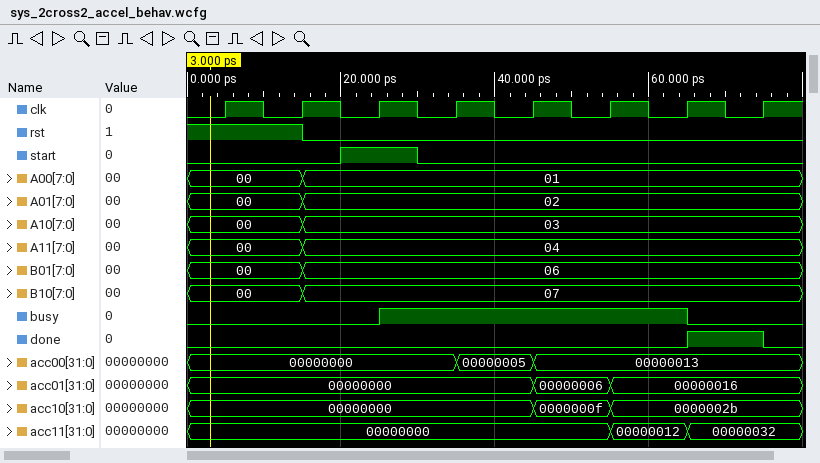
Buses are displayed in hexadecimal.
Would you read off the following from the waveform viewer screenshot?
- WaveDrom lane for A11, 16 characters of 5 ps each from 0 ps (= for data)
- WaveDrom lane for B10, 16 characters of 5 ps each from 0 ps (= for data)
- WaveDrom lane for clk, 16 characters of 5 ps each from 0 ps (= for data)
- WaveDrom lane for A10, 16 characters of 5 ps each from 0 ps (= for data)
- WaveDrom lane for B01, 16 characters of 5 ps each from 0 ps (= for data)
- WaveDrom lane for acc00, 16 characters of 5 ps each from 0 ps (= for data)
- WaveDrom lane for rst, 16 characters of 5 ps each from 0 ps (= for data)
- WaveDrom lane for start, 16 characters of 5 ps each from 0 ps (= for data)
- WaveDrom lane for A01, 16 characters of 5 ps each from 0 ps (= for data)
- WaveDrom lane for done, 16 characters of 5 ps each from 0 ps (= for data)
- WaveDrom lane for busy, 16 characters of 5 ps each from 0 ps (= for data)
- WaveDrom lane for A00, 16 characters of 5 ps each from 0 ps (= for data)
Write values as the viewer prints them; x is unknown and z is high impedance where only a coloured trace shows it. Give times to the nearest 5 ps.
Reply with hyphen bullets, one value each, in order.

- {name: 'A11', wave: '=..=............', data: '00 04'}
- {name: 'B10', wave: '=..=............', data: '00 07'}
- {name: 'clk', wave: '0101010101010101'}
- {name: 'A10', wave: '=..=............', data: '00 03'}
- {name: 'B01', wave: '=..=............', data: '00 06'}
- {name: 'acc00', wave: '=......=.=......', data: '00000000 00000005 00000013'}
- {name: 'rst', wave: '1..0............'}
- {name: 'start', wave: '0...1.0.........'}
- {name: 'A01', wave: '=..=............', data: '00 02'}
- {name: 'done', wave: '0............1.0'}
- {name: 'busy', wave: '0....1.......0..'}
- {name: 'A00', wave: '=..=............', data: '00 01'}
